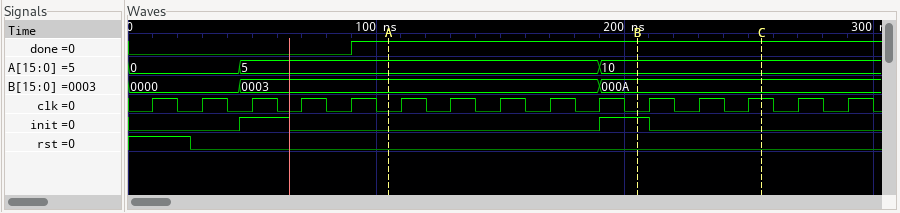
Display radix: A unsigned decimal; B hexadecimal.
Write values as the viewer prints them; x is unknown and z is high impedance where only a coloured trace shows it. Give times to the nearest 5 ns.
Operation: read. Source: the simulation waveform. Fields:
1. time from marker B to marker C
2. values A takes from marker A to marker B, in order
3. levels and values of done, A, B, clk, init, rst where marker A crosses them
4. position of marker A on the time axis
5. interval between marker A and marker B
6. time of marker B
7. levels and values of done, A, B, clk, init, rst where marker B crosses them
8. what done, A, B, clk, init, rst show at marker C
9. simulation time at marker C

50 ns
5, 10
done=1, A=5, B=0003, clk=0, init=0, rst=0
105 ns
100 ns
205 ns
done=1, A=10, B=000A, clk=0, init=1, rst=0
done=1, A=10, B=000A, clk=1, init=0, rst=0
255 ns
